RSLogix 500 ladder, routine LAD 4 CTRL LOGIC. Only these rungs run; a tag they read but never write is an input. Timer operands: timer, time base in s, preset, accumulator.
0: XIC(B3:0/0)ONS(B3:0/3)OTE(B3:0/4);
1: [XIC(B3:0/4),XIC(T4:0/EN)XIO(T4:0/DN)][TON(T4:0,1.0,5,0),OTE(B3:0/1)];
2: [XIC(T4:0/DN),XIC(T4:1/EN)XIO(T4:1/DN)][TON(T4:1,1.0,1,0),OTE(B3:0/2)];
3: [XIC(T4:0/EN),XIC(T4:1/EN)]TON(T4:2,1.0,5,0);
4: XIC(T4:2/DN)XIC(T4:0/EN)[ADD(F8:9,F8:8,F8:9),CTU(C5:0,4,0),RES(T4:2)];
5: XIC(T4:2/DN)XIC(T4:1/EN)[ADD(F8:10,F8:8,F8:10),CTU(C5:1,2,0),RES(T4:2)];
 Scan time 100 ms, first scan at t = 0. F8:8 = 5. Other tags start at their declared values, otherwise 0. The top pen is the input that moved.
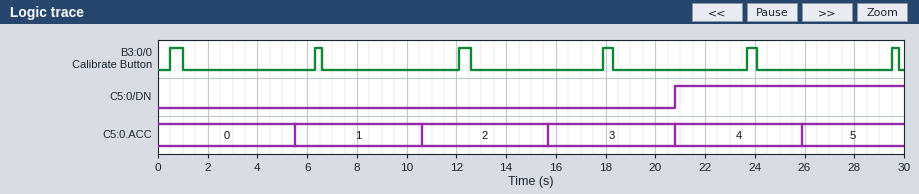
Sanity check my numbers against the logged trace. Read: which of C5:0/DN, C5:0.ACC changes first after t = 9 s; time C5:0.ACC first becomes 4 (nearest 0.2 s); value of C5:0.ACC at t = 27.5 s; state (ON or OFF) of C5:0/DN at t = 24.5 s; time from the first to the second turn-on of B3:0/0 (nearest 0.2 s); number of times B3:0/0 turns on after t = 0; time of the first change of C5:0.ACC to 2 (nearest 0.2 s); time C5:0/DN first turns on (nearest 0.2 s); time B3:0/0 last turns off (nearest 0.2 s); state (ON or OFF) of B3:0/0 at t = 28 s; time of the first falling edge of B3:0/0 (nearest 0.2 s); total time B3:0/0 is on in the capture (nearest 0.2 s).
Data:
C5:0.ACC
20.8 s
5
ON
5.8 s
6
10.6 s
20.8 s
29.8 s
OFF
1.0 s
2.4 s
